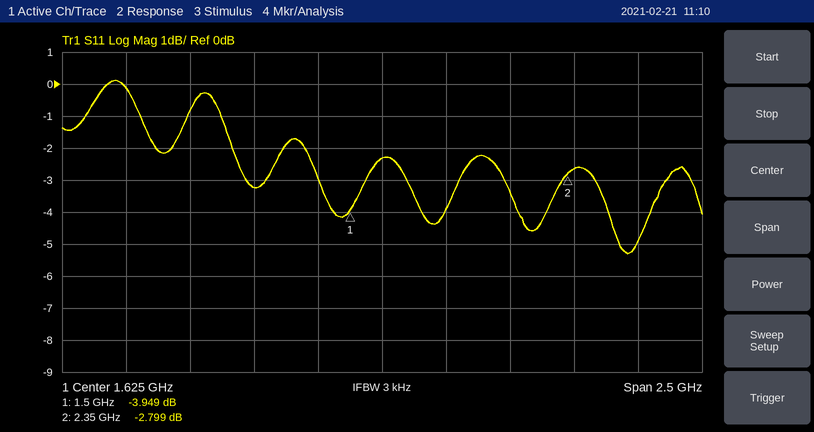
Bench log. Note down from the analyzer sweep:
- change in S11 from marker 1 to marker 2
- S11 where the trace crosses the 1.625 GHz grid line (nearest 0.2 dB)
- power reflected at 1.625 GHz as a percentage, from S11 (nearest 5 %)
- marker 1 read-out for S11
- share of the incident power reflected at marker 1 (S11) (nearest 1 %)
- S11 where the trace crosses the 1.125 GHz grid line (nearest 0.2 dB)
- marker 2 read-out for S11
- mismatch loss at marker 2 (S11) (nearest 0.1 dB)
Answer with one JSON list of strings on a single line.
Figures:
["1.150 dB", "-2.4 dB", "60 %", "-3.949 dB", "40 %", "-3.2 dB", "-2.799 dB", "3.2 dB"]
